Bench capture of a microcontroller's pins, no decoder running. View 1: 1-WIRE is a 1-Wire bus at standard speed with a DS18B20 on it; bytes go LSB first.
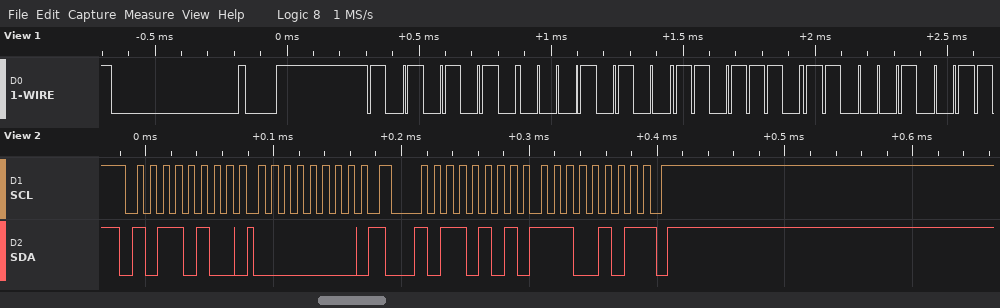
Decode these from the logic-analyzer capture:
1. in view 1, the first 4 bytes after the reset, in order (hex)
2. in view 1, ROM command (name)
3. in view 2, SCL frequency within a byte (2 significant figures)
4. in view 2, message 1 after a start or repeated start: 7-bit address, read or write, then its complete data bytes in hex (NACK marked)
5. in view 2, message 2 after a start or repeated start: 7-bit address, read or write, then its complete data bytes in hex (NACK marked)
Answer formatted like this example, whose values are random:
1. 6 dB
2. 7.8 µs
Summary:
1. 55 28 BB 91
2. Match ROM
3. 100 kHz
4. 0x5A write: 00
5. 0x5A read: E5 NACK
